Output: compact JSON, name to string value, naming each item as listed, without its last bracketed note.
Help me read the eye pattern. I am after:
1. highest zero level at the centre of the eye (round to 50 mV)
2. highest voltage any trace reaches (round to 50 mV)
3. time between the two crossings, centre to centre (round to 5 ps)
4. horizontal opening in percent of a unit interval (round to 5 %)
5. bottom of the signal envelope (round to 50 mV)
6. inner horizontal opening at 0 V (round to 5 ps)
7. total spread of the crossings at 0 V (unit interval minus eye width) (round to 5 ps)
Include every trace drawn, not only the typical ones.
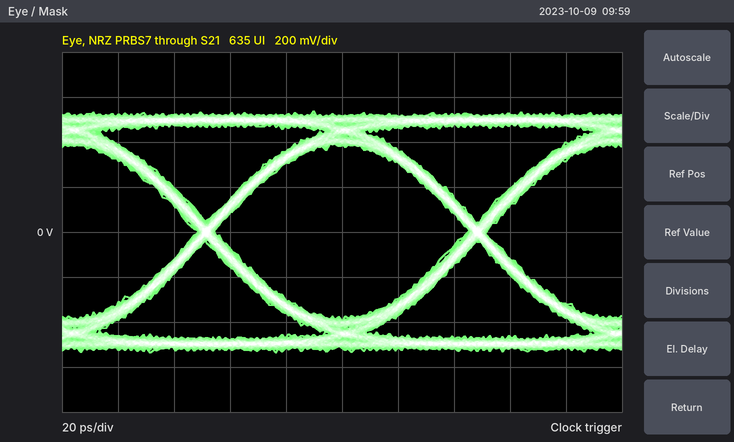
{"highest zero level at the centre of the eye": "-400 mV", "highest voltage any trace reaches": "550 mV", "time between the two crossings, centre to centre": "95 ps", "horizontal opening in percent of a unit interval": "95 %", "bottom of the signal envelope": "-550 mV", "inner horizontal opening at 0 V": "90 ps", "total spread of the crossings at 0 V (unit interval minus eye width)": "5 ps"}
